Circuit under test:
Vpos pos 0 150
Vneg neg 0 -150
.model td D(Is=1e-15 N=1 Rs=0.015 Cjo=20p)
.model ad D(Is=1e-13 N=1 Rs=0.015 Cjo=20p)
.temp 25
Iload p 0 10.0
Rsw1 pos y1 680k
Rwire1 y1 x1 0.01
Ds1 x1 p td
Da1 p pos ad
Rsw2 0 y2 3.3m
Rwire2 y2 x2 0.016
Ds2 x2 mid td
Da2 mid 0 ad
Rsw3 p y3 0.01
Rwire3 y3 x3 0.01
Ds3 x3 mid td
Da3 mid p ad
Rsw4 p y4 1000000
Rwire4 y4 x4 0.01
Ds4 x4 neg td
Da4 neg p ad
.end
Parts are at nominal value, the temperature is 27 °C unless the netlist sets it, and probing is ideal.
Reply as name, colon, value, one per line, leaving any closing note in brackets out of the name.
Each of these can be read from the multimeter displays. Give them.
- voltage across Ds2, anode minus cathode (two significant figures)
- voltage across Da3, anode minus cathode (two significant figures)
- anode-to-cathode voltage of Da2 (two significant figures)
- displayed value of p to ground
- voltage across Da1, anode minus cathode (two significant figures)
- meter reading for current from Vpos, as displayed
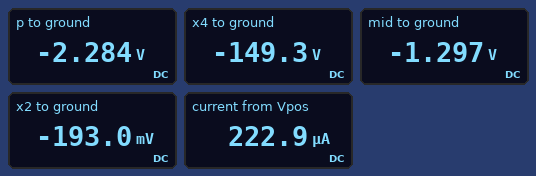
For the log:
voltage across Ds2, anode minus cathode: 1.1 V
voltage across Da3, anode minus cathode: 990 mV
anode-to-cathode voltage of Da2: -1.3 V
displayed value of p to ground: -2.284 V
voltage across Da1, anode minus cathode: -150 V
meter reading for current from Vpos, as displayed: 222.9 µA
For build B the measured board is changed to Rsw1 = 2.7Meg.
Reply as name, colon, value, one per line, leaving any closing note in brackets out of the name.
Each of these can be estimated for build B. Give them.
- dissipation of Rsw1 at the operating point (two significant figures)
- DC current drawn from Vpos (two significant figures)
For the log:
dissipation of Rsw1 at the operating point: 8.5 mW
DC current drawn from Vpos: 56 µA
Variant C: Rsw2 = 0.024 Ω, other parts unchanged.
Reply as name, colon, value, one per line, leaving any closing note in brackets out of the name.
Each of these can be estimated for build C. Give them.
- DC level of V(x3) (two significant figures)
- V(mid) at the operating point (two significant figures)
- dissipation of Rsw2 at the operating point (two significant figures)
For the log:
DC level of V(x3): -2.5 V
V(mid) at the operating point: -1.5 V
dissipation of Rsw2 at the operating point: 2.4 W
